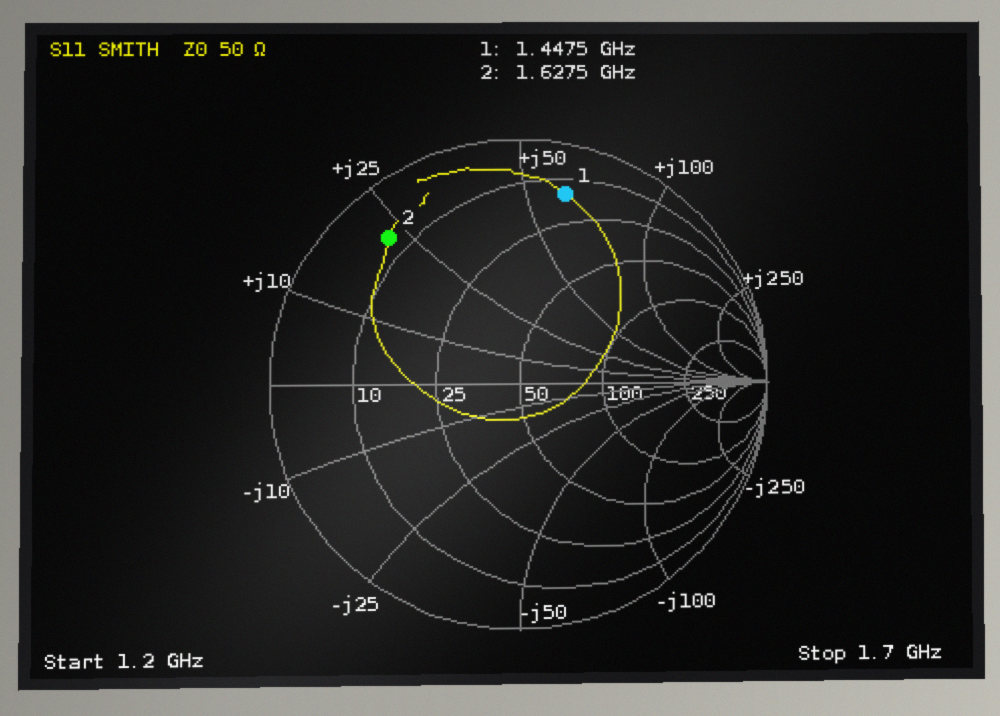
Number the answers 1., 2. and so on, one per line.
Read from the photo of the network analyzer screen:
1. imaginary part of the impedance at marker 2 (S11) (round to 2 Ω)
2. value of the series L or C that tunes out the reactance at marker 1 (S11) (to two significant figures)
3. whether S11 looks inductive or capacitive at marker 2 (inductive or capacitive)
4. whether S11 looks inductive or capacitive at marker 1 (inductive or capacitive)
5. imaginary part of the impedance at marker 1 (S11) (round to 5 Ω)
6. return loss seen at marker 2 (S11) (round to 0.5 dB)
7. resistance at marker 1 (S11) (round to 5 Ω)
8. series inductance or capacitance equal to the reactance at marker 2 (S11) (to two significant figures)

1. +22 Ω
2. 1.8 pF
3. inductive
4. inductive
5. +60 Ω
6. 2.0 dB
7. 15 Ω
8. 2.2 nH
